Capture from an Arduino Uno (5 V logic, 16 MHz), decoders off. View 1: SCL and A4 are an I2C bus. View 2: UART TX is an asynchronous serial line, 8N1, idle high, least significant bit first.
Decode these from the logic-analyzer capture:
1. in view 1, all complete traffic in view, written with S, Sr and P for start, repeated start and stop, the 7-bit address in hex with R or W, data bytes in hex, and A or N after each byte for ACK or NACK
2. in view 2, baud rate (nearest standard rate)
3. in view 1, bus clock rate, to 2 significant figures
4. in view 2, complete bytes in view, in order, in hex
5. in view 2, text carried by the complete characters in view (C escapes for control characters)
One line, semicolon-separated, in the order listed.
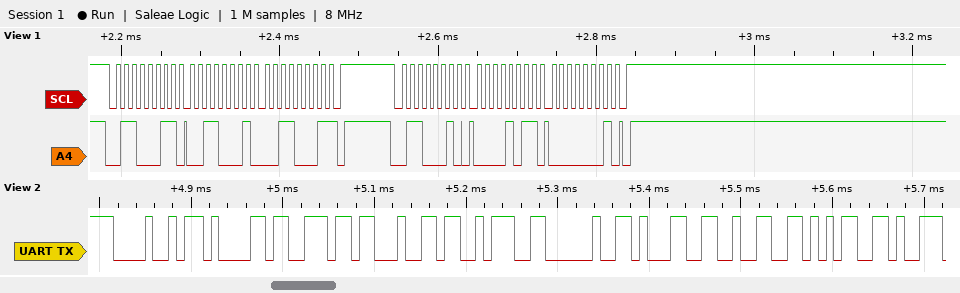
S 31R A 31 A 31 N P S 31W A 0B A 01 A P; 115200 baud; 100 kHz; 0x48 0x61 0x6E 0x64 0x3A 0x20 0x31 0x32 0x35; "Hand: 125"
